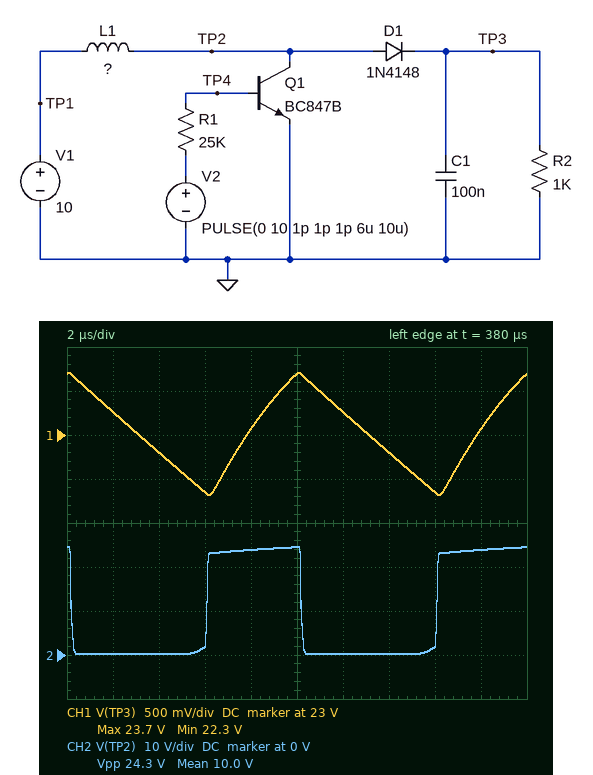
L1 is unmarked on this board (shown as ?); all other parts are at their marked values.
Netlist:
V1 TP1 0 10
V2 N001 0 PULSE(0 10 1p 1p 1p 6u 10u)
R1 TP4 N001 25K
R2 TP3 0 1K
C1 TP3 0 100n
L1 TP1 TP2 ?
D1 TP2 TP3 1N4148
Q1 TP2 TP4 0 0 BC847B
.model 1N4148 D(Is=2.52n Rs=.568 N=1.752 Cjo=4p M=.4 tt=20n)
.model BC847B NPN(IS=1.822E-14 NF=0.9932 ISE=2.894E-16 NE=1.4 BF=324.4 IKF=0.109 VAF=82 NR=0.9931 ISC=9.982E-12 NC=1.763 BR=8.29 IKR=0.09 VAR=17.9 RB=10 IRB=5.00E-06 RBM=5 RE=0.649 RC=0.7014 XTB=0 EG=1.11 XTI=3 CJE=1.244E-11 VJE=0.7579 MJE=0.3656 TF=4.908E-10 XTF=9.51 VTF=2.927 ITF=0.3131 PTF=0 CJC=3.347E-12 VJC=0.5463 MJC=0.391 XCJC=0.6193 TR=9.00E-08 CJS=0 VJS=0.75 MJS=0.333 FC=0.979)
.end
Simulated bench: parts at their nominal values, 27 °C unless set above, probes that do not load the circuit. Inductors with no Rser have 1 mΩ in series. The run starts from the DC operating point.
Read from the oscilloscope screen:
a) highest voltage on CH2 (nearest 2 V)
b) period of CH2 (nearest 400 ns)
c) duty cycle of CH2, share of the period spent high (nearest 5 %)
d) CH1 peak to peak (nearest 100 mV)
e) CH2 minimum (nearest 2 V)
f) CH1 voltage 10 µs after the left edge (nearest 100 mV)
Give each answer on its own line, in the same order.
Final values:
24 V
10.0 µs
40 %
1.4 V
0 V
23.7 V
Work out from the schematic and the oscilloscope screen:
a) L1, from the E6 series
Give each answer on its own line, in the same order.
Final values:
2.2 mH
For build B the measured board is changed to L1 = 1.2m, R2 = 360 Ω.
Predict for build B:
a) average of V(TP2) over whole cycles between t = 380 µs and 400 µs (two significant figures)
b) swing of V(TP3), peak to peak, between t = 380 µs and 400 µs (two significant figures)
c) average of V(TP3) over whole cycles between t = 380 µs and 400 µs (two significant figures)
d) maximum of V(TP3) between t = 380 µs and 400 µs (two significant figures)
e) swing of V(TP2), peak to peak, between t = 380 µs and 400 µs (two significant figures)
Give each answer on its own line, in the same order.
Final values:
10 V
1.7 V
11 V
12 V
6.4 V
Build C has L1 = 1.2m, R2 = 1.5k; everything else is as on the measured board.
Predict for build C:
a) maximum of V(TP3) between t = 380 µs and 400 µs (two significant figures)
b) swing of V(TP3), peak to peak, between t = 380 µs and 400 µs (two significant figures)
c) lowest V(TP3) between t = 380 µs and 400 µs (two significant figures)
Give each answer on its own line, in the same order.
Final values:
25 V
1.0 V
24 V
